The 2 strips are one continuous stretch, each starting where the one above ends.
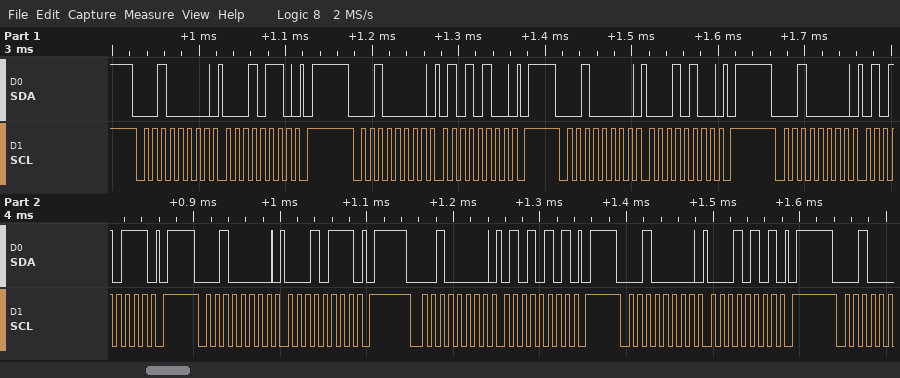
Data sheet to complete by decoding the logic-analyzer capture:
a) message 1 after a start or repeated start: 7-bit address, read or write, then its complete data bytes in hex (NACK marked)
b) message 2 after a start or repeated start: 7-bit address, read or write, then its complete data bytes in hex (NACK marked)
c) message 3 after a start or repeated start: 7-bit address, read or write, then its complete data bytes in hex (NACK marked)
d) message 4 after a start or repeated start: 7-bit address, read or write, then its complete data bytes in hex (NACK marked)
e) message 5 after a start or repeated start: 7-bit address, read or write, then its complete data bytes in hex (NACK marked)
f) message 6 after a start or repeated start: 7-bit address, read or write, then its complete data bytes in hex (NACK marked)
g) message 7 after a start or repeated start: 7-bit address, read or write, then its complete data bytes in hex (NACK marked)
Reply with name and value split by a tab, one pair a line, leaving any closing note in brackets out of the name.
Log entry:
message 1 after a start or repeated start: 7-bit address, read or write, then its complete data bytes in hex	0x10 write: 16
message 2 after a start or repeated start: 7-bit address, read or write, then its complete data bytes in hex	0x10 write: 54
message 3 after a start or repeated start: 7-bit address, read or write, then its complete data bytes in hex	0x10 write: 14
message 4 after a start or repeated start: 7-bit address, read or write, then its complete data bytes in hex	0x10 write: 57
message 5 after a start or repeated start: 7-bit address, read or write, then its complete data bytes in hex	0x10 write: 17
message 6 after a start or repeated start: 7-bit address, read or write, then its complete data bytes in hex	0x10 write: 55
message 7 after a start or repeated start: 7-bit address, read or write, then its complete data bytes in hex	0x10 write: 15
